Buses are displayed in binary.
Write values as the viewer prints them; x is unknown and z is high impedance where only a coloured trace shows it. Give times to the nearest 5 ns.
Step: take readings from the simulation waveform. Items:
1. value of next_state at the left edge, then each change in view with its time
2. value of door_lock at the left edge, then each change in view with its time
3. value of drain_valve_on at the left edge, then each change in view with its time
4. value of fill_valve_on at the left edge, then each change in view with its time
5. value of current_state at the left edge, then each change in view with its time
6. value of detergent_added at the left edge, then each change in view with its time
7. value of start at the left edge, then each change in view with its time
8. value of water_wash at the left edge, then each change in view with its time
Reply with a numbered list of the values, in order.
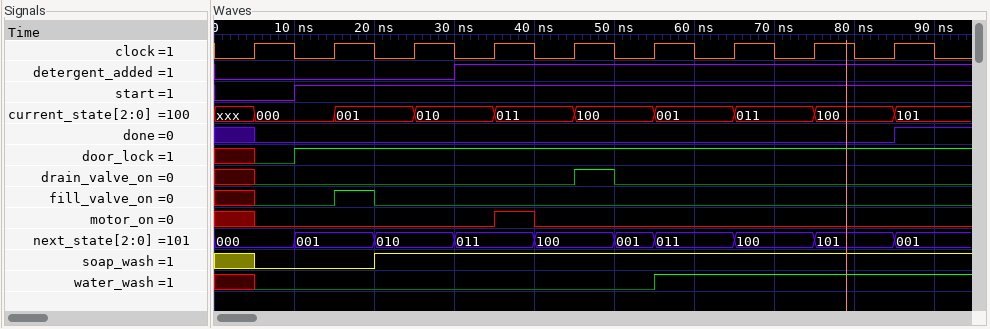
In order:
1. 000, 001 at 10 ns, 010 at 20 ns, 011 at 30 ns, 100 at 40 ns, 001 at 50 ns, 011 at 55 ns, 100 at 65 ns, 101 at 75 ns, 001 at 85 ns
2. x, 0 at 5 ns, 1 at 10 ns
3. x, 0 at 5 ns, 1 at 45 ns, 0 at 50 ns
4. x, 0 at 5 ns, 1 at 15 ns, 0 at 20 ns
5. xxx, 000 at 5 ns, 001 at 15 ns, 010 at 25 ns, 011 at 35 ns, 100 at 45 ns, 001 at 55 ns, 011 at 65 ns, 100 at 75 ns, 101 at 85 ns
6. 0, 1 at 30 ns
7. 0, 1 at 10 ns
8. x, 0 at 5 ns, 1 at 55 ns
